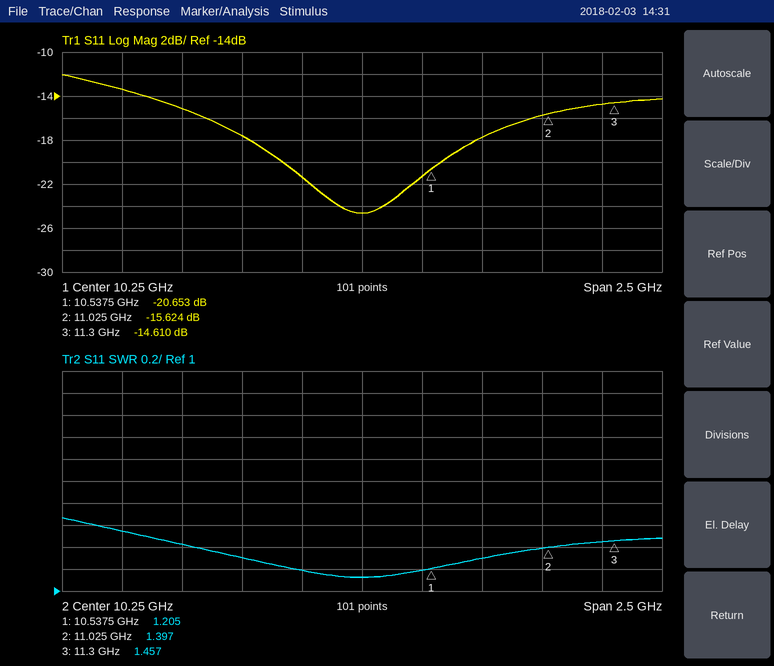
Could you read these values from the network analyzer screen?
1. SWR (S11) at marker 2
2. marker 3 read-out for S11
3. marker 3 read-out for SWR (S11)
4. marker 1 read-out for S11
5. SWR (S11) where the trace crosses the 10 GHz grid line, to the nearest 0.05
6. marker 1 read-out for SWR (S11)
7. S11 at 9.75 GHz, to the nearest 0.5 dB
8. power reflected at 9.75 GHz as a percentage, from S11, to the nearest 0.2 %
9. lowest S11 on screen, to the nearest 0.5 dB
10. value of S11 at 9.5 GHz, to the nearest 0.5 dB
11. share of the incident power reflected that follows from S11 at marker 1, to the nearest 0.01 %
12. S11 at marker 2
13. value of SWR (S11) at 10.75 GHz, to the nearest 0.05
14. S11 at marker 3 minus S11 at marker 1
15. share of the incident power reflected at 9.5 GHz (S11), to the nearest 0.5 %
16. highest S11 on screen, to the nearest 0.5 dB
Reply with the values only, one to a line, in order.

1.397
-14.610 dB
1.457
-20.653 dB
1.20
1.205
-17.5 dB
1.8 %
-24.5 dB
-15.0 dB
0.86 %
-15.624 dB
1.30
6.043 dB
3.0 %
-12.0 dB
